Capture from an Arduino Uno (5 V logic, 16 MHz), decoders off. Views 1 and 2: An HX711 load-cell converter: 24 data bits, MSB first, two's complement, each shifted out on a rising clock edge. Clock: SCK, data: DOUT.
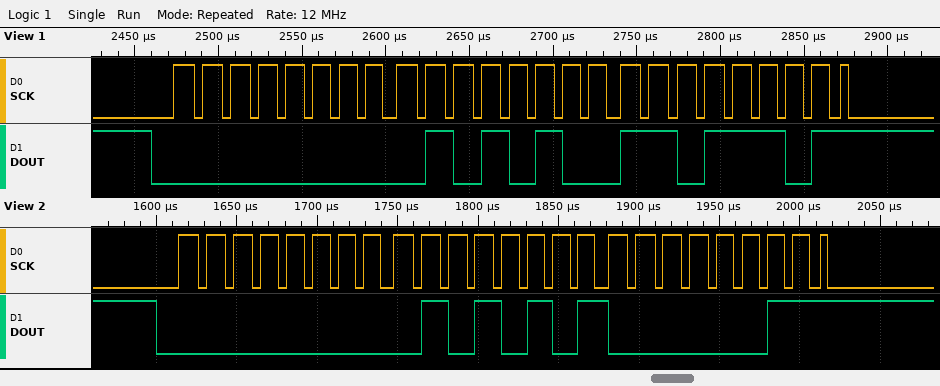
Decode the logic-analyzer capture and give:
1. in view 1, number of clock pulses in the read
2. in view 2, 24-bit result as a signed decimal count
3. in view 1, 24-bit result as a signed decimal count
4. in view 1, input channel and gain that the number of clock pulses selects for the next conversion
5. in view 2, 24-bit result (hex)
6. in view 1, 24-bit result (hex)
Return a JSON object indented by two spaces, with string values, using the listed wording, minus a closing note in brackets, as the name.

{
  "in view 1, number of clock pulses in the read": "25",
  "in view 2, 24-bit result as a signed decimal count": "21763",
  "in view 1, 24-bit result as a signed decimal count": "21725",
  "in view 1, input channel and gain that the number of clock pulses selects for the next conversion": "channel A, gain 128",
  "in view 2, 24-bit result": "0x005503",
  "in view 1, 24-bit result": "0x0054DD"
}
